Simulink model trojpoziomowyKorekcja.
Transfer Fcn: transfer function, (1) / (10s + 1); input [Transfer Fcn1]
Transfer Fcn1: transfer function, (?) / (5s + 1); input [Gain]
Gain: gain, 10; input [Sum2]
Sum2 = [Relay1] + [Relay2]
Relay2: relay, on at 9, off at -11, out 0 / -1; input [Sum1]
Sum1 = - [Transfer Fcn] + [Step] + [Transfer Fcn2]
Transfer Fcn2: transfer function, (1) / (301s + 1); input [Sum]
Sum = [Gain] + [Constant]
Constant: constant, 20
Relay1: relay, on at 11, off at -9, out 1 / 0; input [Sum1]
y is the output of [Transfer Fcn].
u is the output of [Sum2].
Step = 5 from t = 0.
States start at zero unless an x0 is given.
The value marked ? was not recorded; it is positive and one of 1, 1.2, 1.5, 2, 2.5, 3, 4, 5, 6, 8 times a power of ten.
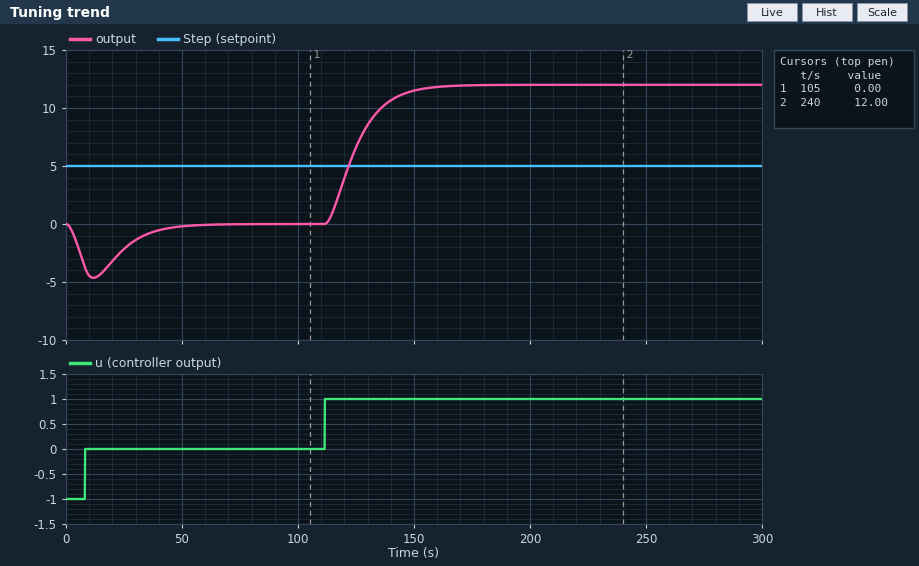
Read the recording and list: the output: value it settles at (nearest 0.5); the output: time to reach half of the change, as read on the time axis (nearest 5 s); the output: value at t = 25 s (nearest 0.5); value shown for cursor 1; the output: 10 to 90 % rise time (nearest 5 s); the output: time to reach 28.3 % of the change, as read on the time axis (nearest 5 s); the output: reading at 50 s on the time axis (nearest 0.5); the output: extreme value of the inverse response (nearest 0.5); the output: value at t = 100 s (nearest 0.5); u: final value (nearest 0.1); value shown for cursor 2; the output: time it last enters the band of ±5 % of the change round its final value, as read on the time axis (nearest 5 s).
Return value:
12.0
125 s
-2.0
0.00
25 s
120 s
0.0
-4.5
0.0
1.0
12.00
150 s
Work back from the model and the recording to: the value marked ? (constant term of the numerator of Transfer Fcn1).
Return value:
1.2
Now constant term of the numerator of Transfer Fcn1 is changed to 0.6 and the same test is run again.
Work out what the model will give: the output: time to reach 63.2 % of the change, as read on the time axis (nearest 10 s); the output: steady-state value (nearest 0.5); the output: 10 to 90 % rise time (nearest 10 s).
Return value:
130 s
6.0
30 s
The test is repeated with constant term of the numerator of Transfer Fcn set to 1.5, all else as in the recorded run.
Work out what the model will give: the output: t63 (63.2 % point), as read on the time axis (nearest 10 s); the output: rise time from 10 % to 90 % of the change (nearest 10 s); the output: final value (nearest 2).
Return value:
130 s
30 s
18
